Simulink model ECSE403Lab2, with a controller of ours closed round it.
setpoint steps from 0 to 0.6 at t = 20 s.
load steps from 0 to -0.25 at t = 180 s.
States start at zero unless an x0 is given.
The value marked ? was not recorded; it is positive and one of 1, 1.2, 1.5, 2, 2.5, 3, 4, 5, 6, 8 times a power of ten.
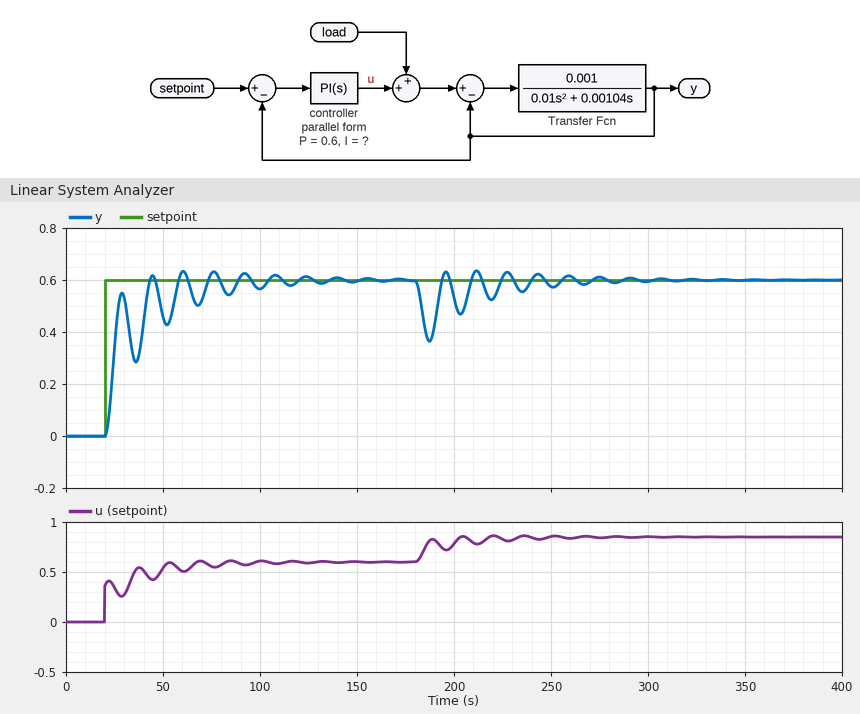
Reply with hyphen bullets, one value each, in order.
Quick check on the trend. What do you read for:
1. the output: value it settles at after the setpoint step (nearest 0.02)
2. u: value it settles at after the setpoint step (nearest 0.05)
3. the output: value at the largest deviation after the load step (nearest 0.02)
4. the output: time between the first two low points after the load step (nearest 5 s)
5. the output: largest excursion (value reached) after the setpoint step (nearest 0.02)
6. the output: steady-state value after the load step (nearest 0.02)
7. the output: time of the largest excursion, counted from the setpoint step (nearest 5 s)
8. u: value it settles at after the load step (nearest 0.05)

- 0.60
- 0.60
- 0.36
- 15 s
- 0.64
- 0.60
- 40 s
- 0.85
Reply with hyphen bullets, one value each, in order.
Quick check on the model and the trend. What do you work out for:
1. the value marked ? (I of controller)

- 0.08
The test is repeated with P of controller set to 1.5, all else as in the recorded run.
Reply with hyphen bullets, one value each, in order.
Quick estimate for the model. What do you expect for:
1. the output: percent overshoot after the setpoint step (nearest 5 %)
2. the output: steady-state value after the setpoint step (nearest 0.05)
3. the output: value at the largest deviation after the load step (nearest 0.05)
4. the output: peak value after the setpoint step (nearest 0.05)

- 15 %
- 0.60
- 0.45
- 0.70
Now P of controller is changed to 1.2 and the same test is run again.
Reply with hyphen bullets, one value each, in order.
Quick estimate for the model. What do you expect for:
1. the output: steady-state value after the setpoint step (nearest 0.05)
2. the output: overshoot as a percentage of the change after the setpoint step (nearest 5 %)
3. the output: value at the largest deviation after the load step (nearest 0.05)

- 0.60
- 10 %
- 0.40
